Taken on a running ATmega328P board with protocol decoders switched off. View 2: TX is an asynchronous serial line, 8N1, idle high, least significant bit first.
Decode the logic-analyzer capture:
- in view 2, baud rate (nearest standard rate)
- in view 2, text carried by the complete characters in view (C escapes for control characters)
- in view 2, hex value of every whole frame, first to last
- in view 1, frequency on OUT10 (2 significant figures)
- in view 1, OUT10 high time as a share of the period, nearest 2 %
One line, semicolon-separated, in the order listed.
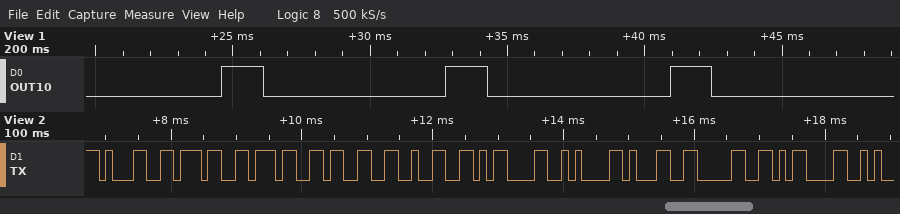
9600 baud; "17732\r\n10\r"; 31 37 37 33 32 0D 0A 31 30 0D; 120 Hz; 18 %
